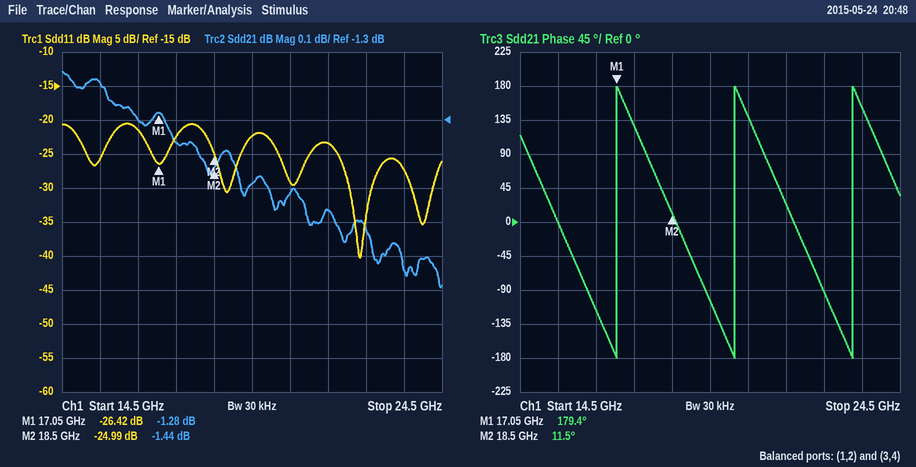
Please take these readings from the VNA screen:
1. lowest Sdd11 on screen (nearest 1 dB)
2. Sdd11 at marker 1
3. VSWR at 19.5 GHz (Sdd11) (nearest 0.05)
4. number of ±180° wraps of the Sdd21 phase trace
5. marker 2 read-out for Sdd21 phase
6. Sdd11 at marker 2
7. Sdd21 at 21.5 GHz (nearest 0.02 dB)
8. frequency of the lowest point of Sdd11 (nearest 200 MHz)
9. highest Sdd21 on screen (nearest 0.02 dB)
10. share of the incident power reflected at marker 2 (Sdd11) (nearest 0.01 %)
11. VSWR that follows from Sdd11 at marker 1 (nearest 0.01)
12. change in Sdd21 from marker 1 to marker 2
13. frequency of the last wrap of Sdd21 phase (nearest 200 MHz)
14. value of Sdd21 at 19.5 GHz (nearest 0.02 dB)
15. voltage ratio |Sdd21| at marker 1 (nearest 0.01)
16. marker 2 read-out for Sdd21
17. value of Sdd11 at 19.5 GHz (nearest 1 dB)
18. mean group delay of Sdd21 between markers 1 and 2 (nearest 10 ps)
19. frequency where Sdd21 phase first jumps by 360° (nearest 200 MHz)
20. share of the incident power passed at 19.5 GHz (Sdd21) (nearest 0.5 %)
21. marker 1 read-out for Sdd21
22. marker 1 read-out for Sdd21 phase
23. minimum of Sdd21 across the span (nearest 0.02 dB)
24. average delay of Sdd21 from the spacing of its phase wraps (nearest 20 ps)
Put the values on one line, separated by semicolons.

-40 dB; -26.42 dB; 1.15; 3; 11.5°; -24.99 dB; -1.56 dB; 22.4 GHz; -1.16 dB; 0.32 %; 1.10; -0.16 dB; 23.2 GHz; -1.48 dB; 0.86; -1.44 dB; -22 dB; 320 ps; 17.0 GHz; 71.0 %; -1.28 dB; 179.4°; -1.80 dB; 320 ps
